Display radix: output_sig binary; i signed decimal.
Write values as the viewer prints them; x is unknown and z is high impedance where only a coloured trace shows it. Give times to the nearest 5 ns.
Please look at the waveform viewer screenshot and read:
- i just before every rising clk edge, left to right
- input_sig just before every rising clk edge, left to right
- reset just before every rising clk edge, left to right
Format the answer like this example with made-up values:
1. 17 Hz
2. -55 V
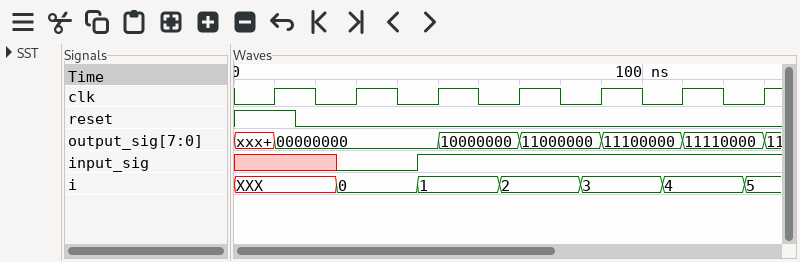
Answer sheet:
1. XXX, 0, 1, 2, 3, 4, 5
2. x 0 1 1 1 1 1
3. 1 0 0 0 0 0 0
